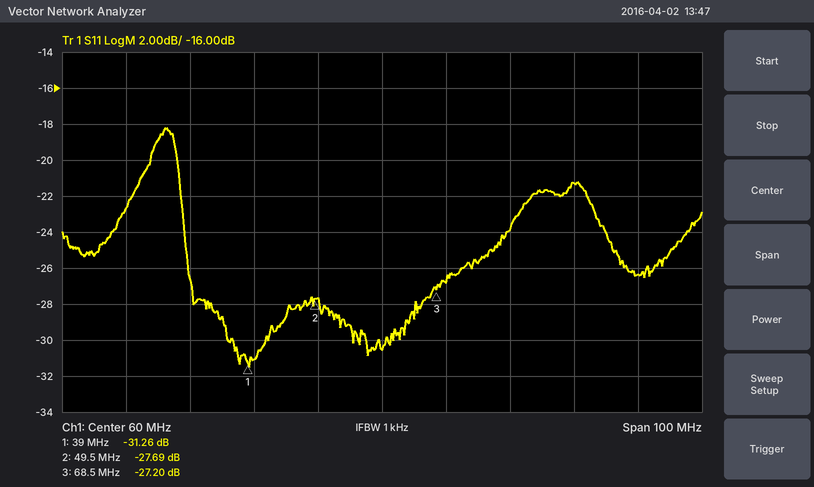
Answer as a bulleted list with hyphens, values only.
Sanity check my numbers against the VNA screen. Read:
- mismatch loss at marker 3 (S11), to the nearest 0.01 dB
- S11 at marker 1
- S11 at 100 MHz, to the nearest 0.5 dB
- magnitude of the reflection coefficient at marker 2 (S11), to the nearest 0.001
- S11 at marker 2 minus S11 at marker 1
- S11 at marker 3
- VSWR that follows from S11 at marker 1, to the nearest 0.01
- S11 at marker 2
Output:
- 0.01 dB
- -31.26 dB
- -26.5 dB
- 0.041
- 3.57 dB
- -27.20 dB
- 1.06
- -27.69 dB
